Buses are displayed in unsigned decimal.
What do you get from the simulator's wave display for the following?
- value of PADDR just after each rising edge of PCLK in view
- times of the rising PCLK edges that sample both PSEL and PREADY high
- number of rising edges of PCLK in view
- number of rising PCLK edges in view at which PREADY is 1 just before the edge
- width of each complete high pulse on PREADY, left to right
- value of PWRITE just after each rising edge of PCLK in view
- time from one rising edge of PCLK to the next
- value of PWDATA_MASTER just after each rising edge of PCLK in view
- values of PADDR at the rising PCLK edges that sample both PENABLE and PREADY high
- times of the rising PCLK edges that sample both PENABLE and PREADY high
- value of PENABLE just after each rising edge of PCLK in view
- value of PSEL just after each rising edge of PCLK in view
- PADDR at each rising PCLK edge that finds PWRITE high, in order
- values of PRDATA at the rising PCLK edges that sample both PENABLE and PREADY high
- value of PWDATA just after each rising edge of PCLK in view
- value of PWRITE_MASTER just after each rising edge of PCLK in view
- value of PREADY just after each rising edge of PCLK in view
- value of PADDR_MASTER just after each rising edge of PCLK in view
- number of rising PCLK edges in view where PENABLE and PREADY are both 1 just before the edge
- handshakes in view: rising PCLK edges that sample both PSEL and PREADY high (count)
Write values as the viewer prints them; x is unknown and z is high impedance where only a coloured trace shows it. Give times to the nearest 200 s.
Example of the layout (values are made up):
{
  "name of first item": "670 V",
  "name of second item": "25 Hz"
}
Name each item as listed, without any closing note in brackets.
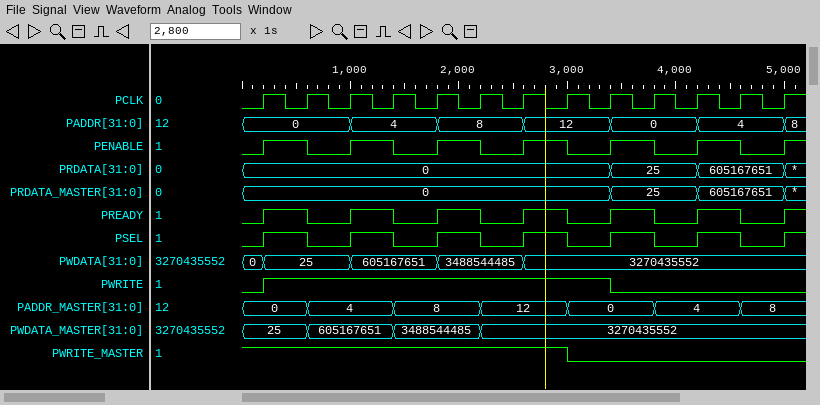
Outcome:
{
  "value of PADDR just after each rising edge of PCLK in view": "0, 0, 4, 4, 8, 8, 12, 12, 0, 0, 4, 4, 8",
  "times of the rising PCLK edges that sample both PSEL and PREADY high": "600 s, 1400 s, 2200 s, 3000 s, 3800 s, 4600 s",
  "number of rising edges of PCLK in view": "13",
  "number of rising PCLK edges in view at which PREADY is 1 just before the edge": "6",
  "width of each complete high pulse on PREADY, left to right": "400 s, 400 s, 400 s, 400 s, 400 s, 400 s",
  "value of PWRITE just after each rising edge of PCLK in view": "1 1 1 1 1 1 1 1 0 0 0 0 0",
  "time from one rising edge of PCLK to the next": "400 s",
  "value of PWDATA_MASTER just after each rising edge of PCLK in view": "25, 605167651, 605167651, 3488544485, 3488544485, 3270435552, 3270435552, 3270435552, 3270435552, 3270435552, 3270435552, 3270435552, 3270435552",
  "values of PADDR at the rising PCLK edges that sample both PENABLE and PREADY high": "0, 4, 8, 12, 0, 4",
  "times of the rising PCLK edges that sample both PENABLE and PREADY high": "600 s, 1400 s, 2200 s, 3000 s, 3800 s, 4600 s",
  "value of PENABLE just after each rising edge of PCLK in view": "1 0 1 0 1 0 1 0 1 0 1 0 1",
  "value of PSEL just after each rising edge of PCLK in view": "1 0 1 0 1 0 1 0 1 0 1 0 1",
  "PADDR at each rising PCLK edge that finds PWRITE high, in order": "0, 0, 4, 4, 8, 8, 12, 12",
  "values of PRDATA at the rising PCLK edges that sample both PENABLE and PREADY high": "0, 0, 0, 0, 25, 605167651",
  "value of PWDATA just after each rising edge of PCLK in view": "25, 25, 605167651, 605167651, 3488544485, 3488544485, 3270435552, 3270435552, 3270435552, 3270435552, 3270435552, 3270435552, 3270435552",
  "value of PWRITE_MASTER just after each rising edge of PCLK in view": "1 1 1 1 1 1 1 0 0 0 0 0 0",
  "value of PREADY just after each rising edge of PCLK in view": "1 0 1 0 1 0 1 0 1 0 1 0 1",
  "value of PADDR_MASTER just after each rising edge of PCLK in view": "0, 4, 4, 8, 8, 12, 12, 0, 0, 4, 4, 8, 8",
  "number of rising PCLK edges in view where PENABLE and PREADY are both 1 just before the edge": "6",
  "handshakes in view: rising PCLK edges that sample both PSEL and PREADY high": "6"
}
